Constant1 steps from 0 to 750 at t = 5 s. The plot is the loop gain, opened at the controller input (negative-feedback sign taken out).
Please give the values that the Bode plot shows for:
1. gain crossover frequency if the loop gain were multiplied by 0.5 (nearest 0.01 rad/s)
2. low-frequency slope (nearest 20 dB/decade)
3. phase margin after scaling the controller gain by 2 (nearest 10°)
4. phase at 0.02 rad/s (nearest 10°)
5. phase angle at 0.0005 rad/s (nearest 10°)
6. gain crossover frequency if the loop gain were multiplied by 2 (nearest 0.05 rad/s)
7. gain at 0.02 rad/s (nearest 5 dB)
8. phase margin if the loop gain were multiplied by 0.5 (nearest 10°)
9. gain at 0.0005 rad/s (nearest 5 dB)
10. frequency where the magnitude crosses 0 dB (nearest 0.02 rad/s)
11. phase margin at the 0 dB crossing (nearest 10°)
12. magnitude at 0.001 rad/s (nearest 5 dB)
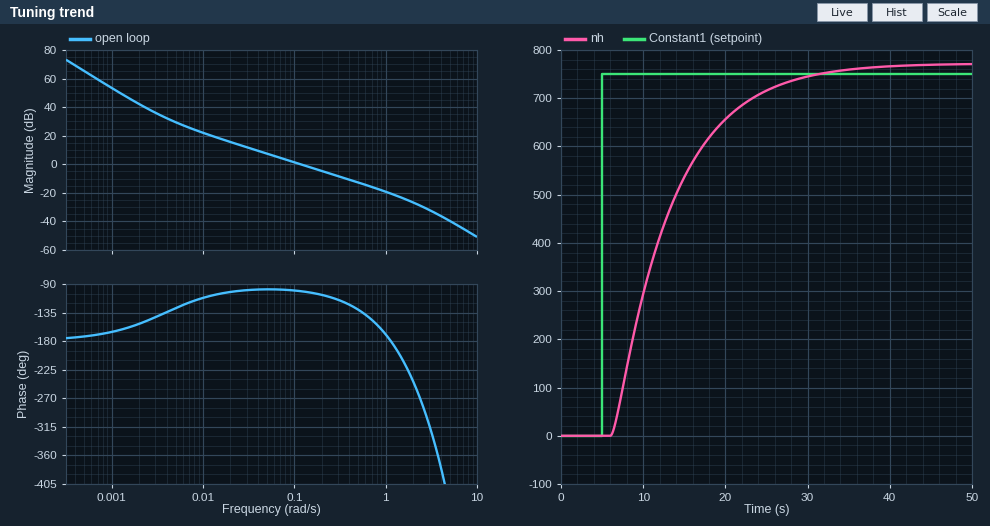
0.06 rad/s
-40 dB/decade
70°
-100°
-170°
0.25 rad/s
15 dB
80°
65 dB
0.12 rad/s
80°
55 dB
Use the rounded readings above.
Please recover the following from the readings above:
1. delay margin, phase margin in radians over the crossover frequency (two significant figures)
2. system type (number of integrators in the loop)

12 s
2
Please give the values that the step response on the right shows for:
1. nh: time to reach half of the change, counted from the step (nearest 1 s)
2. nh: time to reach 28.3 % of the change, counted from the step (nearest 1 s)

6 s
4 s
